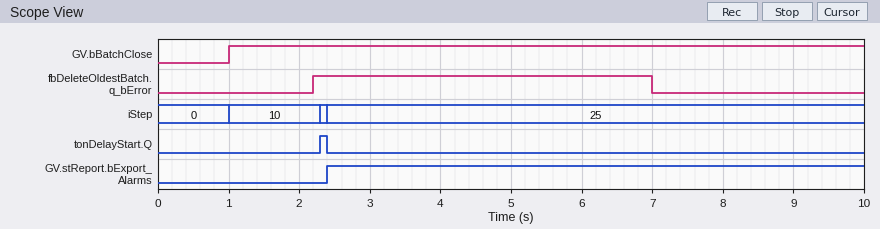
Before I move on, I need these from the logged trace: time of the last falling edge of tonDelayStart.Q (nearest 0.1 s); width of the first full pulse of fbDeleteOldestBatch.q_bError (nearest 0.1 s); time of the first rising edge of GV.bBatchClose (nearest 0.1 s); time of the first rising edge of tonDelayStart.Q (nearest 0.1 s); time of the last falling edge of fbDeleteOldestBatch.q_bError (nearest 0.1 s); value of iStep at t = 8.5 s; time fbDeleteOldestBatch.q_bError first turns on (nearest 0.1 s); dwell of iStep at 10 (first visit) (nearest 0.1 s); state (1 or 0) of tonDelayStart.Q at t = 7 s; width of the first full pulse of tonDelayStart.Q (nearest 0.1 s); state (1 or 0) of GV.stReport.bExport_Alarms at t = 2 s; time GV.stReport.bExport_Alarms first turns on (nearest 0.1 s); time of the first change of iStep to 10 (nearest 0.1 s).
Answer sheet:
2.4 s
4.8 s
1.0 s
2.3 s
7.0 s
25
2.2 s
1.3 s
0
0.1 s
0
2.4 s
1.0 s
